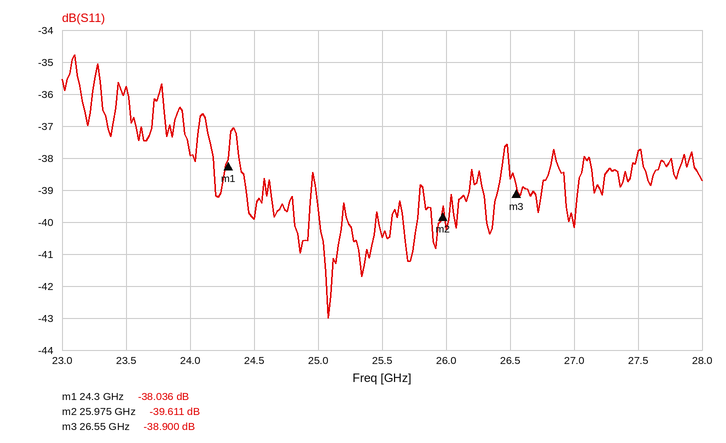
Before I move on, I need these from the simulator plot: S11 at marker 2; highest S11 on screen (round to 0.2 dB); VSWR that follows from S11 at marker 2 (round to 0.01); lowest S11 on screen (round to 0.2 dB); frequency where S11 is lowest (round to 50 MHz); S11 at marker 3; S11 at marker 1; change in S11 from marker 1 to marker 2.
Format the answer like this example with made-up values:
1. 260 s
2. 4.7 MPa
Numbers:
1. -39.611 dB
2. -34.8 dB
3. 1.02
4. -43.0 dB
5. 25.10 GHz
6. -38.900 dB
7. -38.036 dB
8. -1.575 dB
